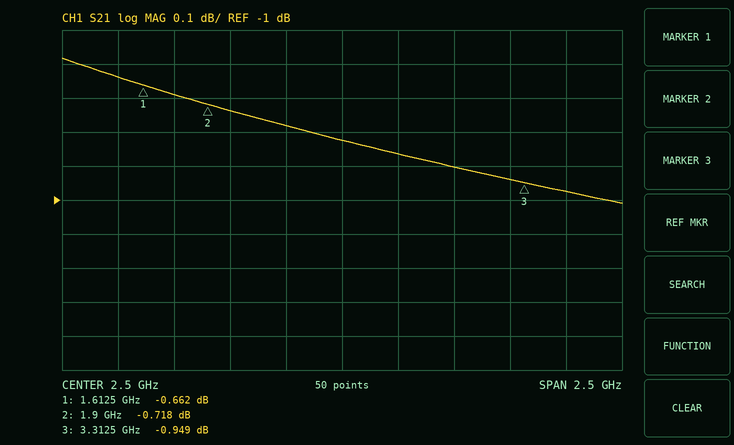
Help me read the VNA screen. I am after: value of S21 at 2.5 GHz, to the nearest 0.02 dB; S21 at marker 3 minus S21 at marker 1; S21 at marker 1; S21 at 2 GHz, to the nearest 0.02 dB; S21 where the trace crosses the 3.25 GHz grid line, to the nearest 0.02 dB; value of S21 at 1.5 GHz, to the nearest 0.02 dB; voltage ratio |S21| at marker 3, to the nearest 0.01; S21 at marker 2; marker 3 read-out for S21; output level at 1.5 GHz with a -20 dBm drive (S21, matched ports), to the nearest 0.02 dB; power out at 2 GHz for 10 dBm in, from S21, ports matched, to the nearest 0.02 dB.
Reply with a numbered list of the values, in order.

1. -0.82 dB
2. -0.287 dB
3. -0.662 dB
4. -0.74 dB
5. -0.94 dB
6. -0.64 dB
7. 0.90
8. -0.718 dB
9. -0.949 dB
10. -20.64 dBm
11. 9.26 dBm
